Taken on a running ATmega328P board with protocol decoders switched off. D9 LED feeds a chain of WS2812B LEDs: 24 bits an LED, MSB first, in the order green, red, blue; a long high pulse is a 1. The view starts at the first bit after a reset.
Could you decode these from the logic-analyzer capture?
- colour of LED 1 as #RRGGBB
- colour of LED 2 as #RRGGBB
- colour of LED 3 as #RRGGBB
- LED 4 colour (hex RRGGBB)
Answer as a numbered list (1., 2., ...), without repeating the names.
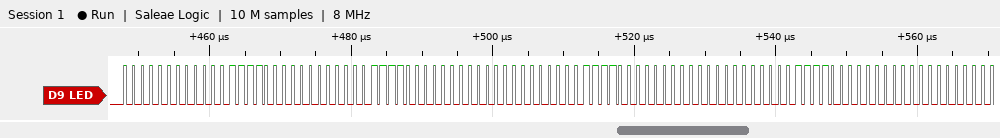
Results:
1. #0F0000
2. #000F00
3. #000F00
4. #000F00
